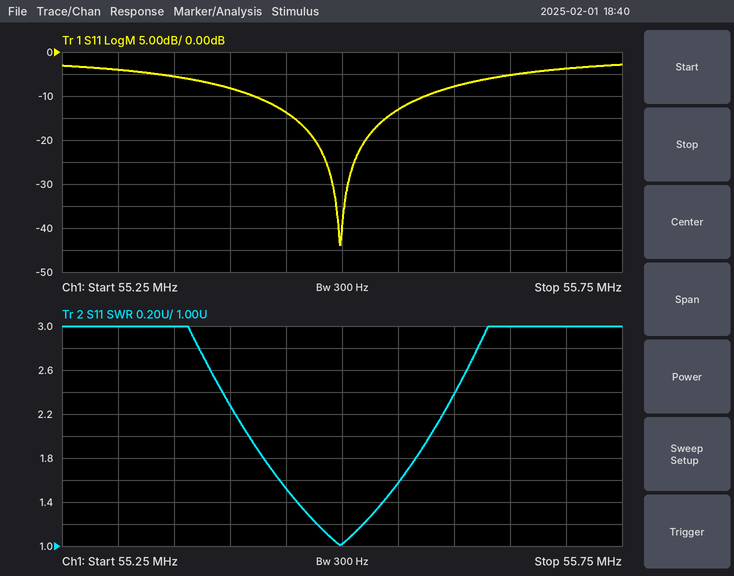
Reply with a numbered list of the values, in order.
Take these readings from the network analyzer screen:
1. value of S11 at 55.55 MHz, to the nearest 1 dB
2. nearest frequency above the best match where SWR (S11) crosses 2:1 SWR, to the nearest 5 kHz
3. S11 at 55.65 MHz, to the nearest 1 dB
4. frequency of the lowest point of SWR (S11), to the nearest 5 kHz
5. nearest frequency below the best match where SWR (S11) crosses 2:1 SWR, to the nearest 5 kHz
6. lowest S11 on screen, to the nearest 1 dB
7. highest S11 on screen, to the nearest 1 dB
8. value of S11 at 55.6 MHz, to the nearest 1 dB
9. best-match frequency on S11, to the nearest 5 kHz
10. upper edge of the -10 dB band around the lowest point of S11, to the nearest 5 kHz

1. -13 dB
2. 55.580 MHz
3. -5 dB
4. 55.500 MHz
5. 55.415 MHz
6. -44 dB
7. -3 dB
8. -8 dB
9. 55.500 MHz
10. 55.575 MHz
